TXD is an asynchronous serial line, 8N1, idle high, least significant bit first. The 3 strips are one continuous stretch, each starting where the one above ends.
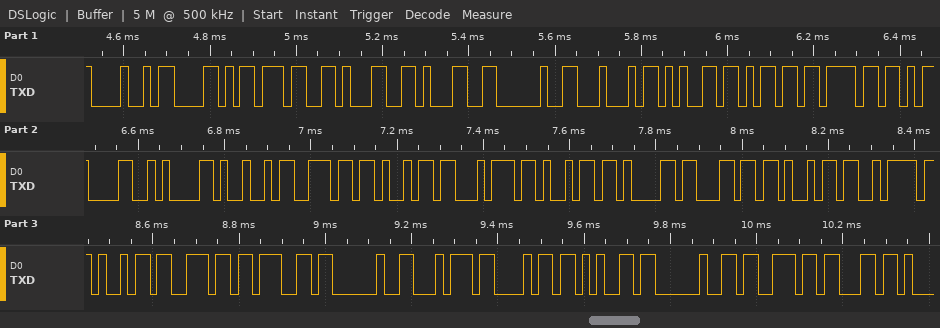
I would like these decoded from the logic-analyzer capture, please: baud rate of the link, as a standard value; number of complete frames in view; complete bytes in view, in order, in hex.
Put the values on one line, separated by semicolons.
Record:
57600 baud; 31; 48 58 37 31 31 20 44 65 6D 6F 0D 0A 49 6E 69 74 69 61 6C 69 7A 69 6E 67 20 74 68 65 20 73 63
